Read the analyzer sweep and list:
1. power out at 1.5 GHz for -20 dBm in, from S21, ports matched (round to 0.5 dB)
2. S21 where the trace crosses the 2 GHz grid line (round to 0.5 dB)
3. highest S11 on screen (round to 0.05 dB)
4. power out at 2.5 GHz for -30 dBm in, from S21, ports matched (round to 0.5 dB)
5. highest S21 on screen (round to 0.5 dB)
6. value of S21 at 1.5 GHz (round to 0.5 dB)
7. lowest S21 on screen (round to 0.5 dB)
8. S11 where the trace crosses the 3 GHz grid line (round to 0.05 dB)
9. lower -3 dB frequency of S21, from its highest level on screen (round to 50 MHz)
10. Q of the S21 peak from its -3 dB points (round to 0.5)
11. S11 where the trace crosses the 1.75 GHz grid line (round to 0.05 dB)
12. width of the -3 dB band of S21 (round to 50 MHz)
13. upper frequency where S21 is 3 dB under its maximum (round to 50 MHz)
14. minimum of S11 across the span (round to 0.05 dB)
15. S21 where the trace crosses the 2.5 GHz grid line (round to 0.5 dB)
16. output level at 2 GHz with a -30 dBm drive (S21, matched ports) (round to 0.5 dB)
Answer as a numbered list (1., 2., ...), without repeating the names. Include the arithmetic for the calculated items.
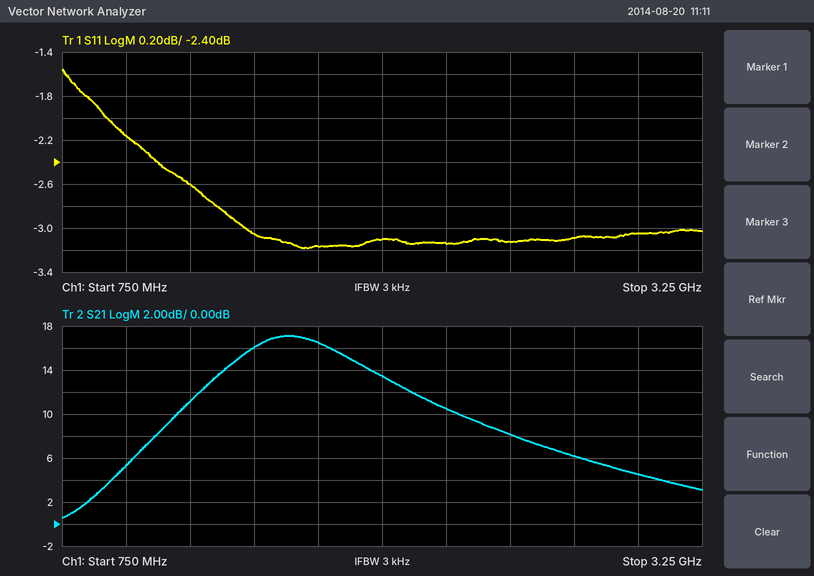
1. -20 dBm + (16.0 dB) = -4.0 dBm
2. 13.5 dB
3. -1.55 dB
4. -30 dBm + (8.0 dB) = -22.0 dBm
5. 17.0 dB
6. 16.0 dB
7. 0.5 dB
8. -3.05 dB
9. 1.40 GHz
10. 1.675 GHz / 550 MHz ≈ 3.0
11. -3.15 dB
12. 1.95 GHz − 1.40 GHz = 550 MHz
13. 1.95 GHz
14. -3.20 dB
15. 8.0 dB
16. -30 dBm + (13.5 dB) = -16.5 dBm
